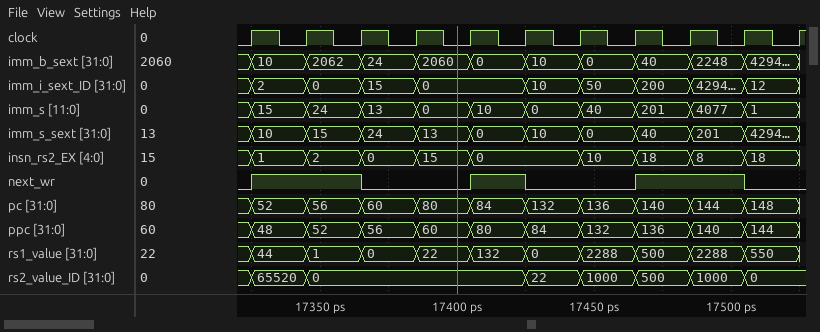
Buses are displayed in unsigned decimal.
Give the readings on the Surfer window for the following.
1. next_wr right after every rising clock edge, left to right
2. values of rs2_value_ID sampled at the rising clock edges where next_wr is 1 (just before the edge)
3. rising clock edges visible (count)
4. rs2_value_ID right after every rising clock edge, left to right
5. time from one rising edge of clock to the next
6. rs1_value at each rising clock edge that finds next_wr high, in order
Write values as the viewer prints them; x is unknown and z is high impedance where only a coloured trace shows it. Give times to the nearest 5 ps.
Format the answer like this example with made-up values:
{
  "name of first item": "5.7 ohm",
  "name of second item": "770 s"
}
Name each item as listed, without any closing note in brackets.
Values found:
{
  "next_wr right after every rising clock edge, left to right": "1 1 0 0 1 0 0 1 1 0 0",
  "values of rs2_value_ID sampled at the rising clock edges where next_wr is 1": "65520, 0, 0, 500, 1000",
  "rising clock edges visible": "11",
  "rs2_value_ID right after every rising clock edge, left to right": "65520, 0, 0, 0, 0, 22, 1000, 500, 1000, 0, 0",
  "time from one rising edge of clock to the next": "20 ps",
  "rs1_value at each rising clock edge that finds next_wr high, in order": "44, 1, 132, 500, 2288"
}
